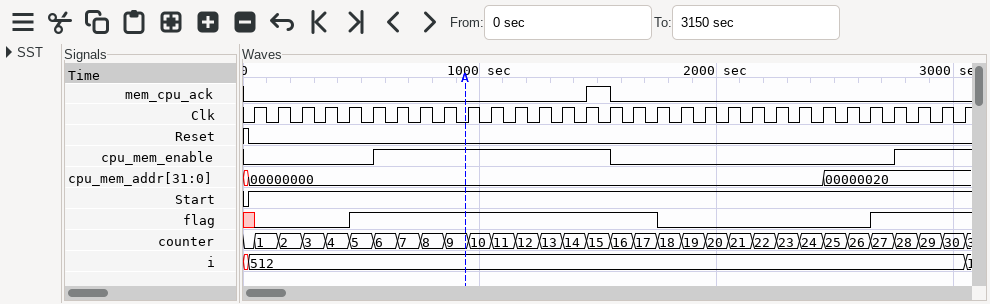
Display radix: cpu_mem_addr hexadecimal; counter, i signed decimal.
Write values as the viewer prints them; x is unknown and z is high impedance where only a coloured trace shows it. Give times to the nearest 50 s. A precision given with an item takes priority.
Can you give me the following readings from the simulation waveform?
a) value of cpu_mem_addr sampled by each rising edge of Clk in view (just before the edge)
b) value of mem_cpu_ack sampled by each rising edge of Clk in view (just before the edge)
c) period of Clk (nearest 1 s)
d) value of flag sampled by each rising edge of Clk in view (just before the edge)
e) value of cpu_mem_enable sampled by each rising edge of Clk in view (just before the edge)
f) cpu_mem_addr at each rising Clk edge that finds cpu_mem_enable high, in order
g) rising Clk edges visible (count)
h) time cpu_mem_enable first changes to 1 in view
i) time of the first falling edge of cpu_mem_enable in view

00000000, 00000000, 00000000, 00000000, 00000000, 00000000, 00000000, 00000000, 00000000, 00000000, 00000000, 00000000, 00000000, 00000000, 00000000, 00000000, 00000000, 00000000, 00000000, 00000000, 00000000, 00000000, 00000000, 00000000, 00000000, 00000020, 00000020, 00000020, 00000020, 00000020, 00000020
0 0 0 0 0 0 0 0 0 0 0 0 0 0 0 1 0 0 0 0 0 0 0 0 0 0 0 0 0 0 0
100 s
x 0 0 0 0 1 1 1 1 1 1 1 1 1 1 1 1 1 0 0 0 0 0 0 0 0 0 1 1 1 1
0 0 0 0 0 0 1 1 1 1 1 1 1 1 1 1 0 0 0 0 0 0 0 0 0 0 0 0 1 1 1
00000000, 00000000, 00000000, 00000000, 00000000, 00000000, 00000000, 00000000, 00000000, 00000000, 00000020, 00000020, 00000020
31
550 s
1550 s
